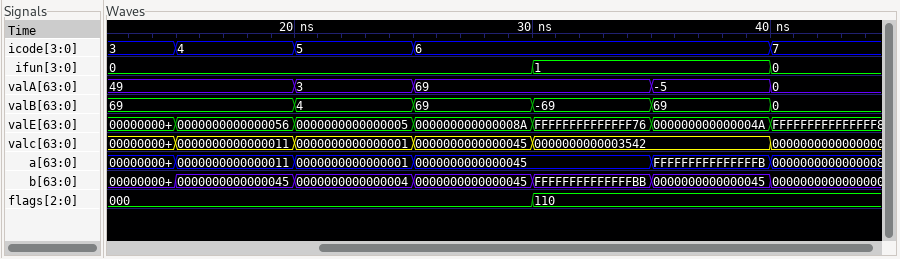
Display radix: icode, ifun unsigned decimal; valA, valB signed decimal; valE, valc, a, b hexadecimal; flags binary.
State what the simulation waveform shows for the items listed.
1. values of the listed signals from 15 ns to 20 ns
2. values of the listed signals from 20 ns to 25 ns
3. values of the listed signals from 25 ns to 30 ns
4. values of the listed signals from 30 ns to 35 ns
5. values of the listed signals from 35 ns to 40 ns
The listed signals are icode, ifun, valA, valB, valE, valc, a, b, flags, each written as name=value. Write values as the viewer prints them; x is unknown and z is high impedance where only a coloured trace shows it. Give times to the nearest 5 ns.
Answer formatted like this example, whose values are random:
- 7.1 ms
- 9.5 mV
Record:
- icode=4, ifun=0, valA=49, valB=69, valE=0000000000000056, valc=0000000000000011, a=0000000000000011, b=0000000000000045, flags=000
- icode=5, ifun=0, valA=3, valB=4, valE=0000000000000005, valc=0000000000000001, a=0000000000000001, b=0000000000000004, flags=000
- icode=6, ifun=0, valA=69, valB=69, valE=000000000000008A, valc=0000000000000045, a=0000000000000045, b=0000000000000045, flags=000
- icode=6, ifun=1, valA=69, valB=-69, valE=FFFFFFFFFFFFFF76, valc=0000000000003542, a=0000000000000045, b=FFFFFFFFFFFFFFBB, flags=110
- icode=6, ifun=1, valA=-5, valB=69, valE=000000000000004A, valc=0000000000003542, a=FFFFFFFFFFFFFFFB, b=0000000000000045, flags=110
